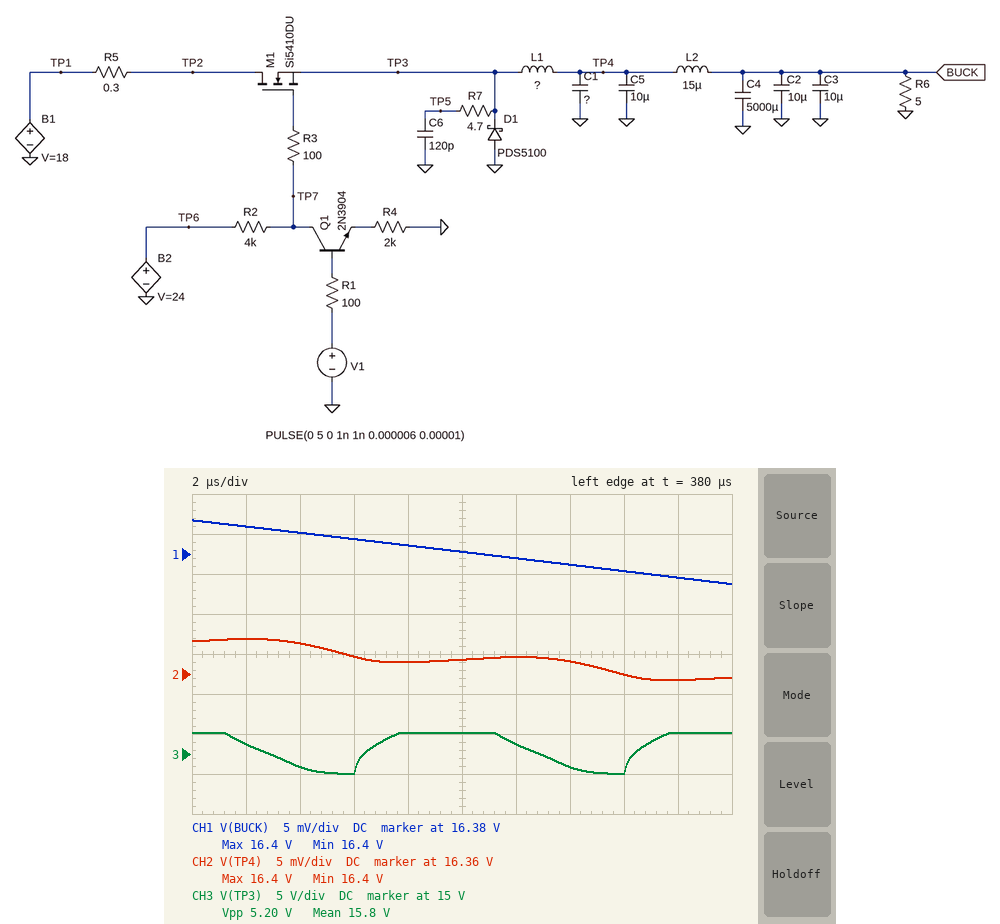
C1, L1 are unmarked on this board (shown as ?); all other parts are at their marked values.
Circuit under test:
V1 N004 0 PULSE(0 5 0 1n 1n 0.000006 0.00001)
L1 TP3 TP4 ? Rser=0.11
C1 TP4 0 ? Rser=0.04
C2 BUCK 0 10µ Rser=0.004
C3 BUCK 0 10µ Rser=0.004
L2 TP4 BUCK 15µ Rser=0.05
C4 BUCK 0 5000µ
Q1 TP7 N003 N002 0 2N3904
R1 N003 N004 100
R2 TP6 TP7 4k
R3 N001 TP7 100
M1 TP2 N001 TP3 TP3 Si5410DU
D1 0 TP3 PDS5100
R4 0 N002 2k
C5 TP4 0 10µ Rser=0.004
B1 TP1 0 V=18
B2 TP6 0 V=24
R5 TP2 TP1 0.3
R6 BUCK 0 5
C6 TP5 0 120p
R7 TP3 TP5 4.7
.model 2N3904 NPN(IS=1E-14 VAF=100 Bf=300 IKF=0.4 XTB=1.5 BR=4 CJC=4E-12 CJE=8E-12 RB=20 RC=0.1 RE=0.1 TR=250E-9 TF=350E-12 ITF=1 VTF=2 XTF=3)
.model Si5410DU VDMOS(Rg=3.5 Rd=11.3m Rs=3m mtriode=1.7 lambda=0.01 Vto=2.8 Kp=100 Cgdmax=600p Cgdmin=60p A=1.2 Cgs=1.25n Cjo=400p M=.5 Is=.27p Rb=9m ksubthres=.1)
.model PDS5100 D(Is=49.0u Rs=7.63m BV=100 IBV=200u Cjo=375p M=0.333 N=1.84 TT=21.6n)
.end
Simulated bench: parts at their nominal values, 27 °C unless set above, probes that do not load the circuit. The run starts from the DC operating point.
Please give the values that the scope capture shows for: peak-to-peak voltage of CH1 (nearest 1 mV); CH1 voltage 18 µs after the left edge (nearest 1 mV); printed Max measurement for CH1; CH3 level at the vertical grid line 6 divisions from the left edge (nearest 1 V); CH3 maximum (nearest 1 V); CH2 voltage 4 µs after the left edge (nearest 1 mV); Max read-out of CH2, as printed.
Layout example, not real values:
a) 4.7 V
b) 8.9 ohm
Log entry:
a) 8 mV
b) 16.372 V
c) 16.4 V
d) 16 V
e) 18 V
f) 16.364 V
g) 16.4 V
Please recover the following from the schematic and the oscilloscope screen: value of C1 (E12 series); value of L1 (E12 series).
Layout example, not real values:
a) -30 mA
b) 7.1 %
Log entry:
a) 680 µF
b) 180 µH
